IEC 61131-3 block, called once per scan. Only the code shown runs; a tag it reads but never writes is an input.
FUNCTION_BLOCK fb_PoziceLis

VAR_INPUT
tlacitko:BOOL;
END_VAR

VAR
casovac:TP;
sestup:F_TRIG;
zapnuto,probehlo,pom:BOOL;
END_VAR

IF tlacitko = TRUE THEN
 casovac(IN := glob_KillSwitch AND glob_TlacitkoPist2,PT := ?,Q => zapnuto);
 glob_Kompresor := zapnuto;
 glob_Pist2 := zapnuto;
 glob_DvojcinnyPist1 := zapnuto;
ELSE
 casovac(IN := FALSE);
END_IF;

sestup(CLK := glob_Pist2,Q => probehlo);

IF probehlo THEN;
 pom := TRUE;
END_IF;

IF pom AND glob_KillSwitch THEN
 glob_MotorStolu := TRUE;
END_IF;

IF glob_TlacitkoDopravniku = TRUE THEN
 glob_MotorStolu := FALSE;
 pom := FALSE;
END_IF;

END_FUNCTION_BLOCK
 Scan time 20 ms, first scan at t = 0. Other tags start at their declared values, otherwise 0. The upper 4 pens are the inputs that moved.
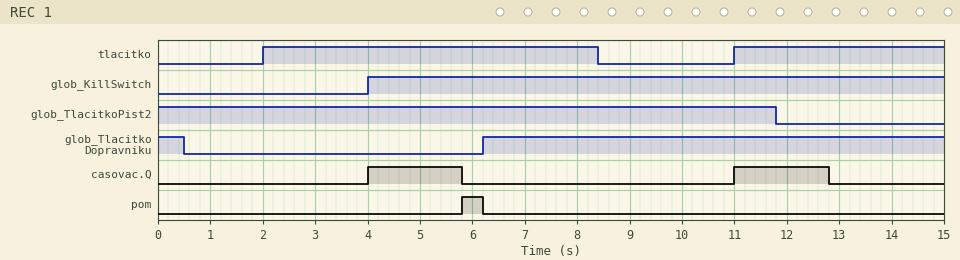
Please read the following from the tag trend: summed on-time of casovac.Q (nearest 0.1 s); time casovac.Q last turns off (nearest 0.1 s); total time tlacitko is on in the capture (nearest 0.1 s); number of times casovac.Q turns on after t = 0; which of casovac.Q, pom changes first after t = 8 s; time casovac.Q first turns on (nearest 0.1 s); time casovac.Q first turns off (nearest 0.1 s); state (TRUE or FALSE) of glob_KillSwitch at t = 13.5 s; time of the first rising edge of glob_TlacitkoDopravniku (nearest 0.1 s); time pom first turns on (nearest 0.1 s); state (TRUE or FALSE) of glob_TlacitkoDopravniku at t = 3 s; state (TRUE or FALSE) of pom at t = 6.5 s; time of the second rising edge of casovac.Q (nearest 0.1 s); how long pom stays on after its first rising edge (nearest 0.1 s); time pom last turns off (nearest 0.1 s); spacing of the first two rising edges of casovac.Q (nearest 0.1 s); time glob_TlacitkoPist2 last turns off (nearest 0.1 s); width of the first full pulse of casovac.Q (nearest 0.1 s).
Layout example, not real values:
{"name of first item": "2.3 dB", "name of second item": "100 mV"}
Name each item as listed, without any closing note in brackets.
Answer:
{"summed on-time of casovac.Q": "3.6 s", "time casovac.Q last turns off": "12.8 s", "total time tlacitko is on in the capture": "10.4 s", "number of times casovac.Q turns on after t = 0": "2", "which of casovac.Q, pom changes first after t = 8 s": "casovac.Q", "time casovac.Q first turns on": "4.0 s", "time casovac.Q first turns off": "5.8 s", "state (TRUE or FALSE) of glob_KillSwitch at t = 13.5 s": "TRUE", "time of the first rising edge of glob_TlacitkoDopravniku": "6.2 s", "time pom first turns on": "5.8 s", "state (TRUE or FALSE) of glob_TlacitkoDopravniku at t = 3 s": "FALSE", "state (TRUE or FALSE) of pom at t = 6.5 s": "FALSE", "time of the second rising edge of casovac.Q": "11.0 s", "how long pom stays on after its first rising edge": "0.4 s", "time pom last turns off": "6.2 s", "spacing of the first two rising edges of casovac.Q": "7.0 s", "time glob_TlacitkoPist2 last turns off": "11.8 s", "width of the first full pulse of casovac.Q": "1.8 s"}
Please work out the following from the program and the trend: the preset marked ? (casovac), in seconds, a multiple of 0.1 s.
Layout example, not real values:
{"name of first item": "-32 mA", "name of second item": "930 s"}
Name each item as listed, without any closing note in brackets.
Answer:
{"the preset marked ? (casovac), in seconds, a multiple of 0.1 s": "1.8 s"}
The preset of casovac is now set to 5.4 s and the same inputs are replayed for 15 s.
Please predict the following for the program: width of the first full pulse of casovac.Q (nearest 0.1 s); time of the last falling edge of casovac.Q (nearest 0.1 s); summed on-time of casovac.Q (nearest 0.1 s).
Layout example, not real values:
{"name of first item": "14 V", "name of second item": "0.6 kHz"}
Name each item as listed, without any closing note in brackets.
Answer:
{"width of the first full pulse of casovac.Q": "5.4 s", "time of the last falling edge of casovac.Q": "9.4 s", "summed on-time of casovac.Q": "9.4 s"}
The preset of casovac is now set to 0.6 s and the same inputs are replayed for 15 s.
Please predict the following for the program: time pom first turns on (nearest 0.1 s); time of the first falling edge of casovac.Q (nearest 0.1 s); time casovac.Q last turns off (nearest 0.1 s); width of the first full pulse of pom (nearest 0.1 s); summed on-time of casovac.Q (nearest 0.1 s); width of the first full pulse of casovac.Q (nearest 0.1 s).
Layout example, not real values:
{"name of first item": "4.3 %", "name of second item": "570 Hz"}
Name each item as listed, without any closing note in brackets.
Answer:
{"time pom first turns on": "4.6 s", "time of the first falling edge of casovac.Q": "4.6 s", "time casovac.Q last turns off": "11.6 s", "width of the first full pulse of pom": "1.6 s", "summed on-time of casovac.Q": "1.2 s", "width of the first full pulse of casovac.Q": "0.6 s"}
